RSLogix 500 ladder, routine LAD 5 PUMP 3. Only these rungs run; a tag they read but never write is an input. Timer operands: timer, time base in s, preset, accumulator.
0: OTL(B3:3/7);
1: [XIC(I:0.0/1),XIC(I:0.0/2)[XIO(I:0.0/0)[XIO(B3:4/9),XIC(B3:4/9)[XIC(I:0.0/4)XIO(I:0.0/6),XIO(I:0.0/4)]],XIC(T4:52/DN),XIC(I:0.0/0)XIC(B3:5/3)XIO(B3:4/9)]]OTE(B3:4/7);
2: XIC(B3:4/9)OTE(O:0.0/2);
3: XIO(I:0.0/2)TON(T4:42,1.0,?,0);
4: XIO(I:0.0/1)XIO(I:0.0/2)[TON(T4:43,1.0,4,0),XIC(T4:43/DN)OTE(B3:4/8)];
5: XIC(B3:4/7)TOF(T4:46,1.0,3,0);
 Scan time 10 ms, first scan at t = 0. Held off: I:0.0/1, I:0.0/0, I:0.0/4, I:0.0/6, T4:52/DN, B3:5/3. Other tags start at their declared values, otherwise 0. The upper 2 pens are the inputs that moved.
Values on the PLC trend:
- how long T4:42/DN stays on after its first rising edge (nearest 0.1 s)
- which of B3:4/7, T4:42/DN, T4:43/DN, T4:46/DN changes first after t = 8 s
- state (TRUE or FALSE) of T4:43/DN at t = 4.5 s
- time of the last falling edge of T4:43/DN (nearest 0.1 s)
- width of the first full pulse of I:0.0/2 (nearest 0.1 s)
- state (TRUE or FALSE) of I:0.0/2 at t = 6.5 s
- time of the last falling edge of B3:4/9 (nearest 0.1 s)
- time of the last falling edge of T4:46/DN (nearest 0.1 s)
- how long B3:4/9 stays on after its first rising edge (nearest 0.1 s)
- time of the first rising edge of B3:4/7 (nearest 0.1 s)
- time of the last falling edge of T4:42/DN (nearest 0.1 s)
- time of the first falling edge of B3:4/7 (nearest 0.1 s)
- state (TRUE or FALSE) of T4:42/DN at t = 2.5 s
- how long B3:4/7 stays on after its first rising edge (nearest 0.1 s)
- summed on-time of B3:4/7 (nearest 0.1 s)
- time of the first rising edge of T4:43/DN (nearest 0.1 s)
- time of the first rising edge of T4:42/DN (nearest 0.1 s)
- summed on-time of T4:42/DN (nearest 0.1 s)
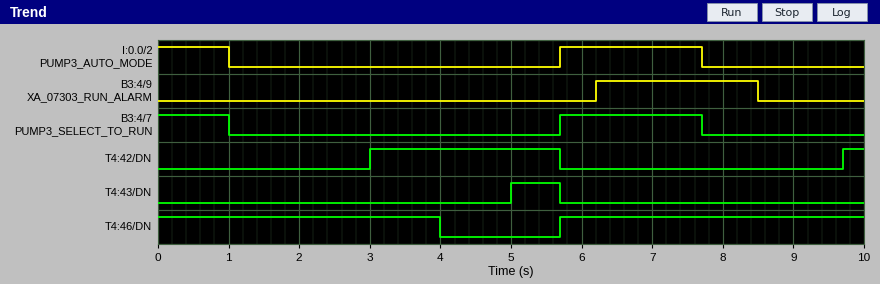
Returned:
2.7 s
T4:42/DN
FALSE
5.7 s
2.0 s
TRUE
8.5 s
4.0 s
2.3 s
5.7 s
5.7 s
1.0 s
FALSE
2.0 s
3.0 s
5.0 s
3.0 s
3.0 s
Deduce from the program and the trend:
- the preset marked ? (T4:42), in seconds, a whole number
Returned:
2 s
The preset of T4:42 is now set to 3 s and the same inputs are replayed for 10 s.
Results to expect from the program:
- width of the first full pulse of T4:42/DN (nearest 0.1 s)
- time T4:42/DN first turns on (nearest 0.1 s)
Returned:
1.7 s
4.0 s
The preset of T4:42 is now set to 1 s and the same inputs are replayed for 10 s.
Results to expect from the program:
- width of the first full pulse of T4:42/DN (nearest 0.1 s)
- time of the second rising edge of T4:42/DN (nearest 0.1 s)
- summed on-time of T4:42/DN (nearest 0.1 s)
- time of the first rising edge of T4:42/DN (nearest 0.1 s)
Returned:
3.7 s
8.7 s
5.0 s
2.0 s
